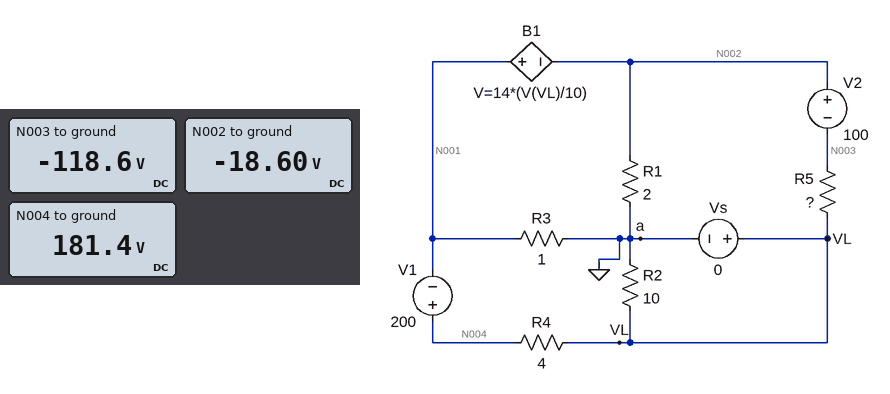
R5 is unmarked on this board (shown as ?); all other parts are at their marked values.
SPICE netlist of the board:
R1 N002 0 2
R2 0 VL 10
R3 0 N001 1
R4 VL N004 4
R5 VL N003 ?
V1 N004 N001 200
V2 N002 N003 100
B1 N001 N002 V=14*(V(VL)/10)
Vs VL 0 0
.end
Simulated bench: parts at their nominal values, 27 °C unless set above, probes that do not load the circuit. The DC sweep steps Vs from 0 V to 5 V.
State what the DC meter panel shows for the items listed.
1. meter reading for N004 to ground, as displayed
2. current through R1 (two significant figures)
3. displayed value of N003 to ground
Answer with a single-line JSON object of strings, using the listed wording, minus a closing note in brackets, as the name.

{"meter reading for N004 to ground, as displayed": "181.4 V", "current through R1": "9.3 A", "displayed value of N003 to ground": "-118.6 V"}
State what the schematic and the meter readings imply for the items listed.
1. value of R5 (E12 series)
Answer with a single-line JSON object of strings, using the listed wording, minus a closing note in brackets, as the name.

{"value of R5": "6.8 Ω"}
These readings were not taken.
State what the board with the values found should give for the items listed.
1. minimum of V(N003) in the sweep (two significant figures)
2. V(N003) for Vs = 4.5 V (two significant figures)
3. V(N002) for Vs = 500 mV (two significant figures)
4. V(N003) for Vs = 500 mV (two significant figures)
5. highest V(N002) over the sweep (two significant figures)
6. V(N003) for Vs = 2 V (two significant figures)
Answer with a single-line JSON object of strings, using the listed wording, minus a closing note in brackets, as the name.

{"minimum of V(N003) in the sweep": "-120 V", "V(N003) for Vs = 4.5 V": "-120 V", "V(N002) for Vs = 500 mV": "-19 V", "V(N003) for Vs = 500 mV": "-120 V", "highest V(N002) over the sweep": "-19 V", "V(N003) for Vs = 2 V": "-120 V"}
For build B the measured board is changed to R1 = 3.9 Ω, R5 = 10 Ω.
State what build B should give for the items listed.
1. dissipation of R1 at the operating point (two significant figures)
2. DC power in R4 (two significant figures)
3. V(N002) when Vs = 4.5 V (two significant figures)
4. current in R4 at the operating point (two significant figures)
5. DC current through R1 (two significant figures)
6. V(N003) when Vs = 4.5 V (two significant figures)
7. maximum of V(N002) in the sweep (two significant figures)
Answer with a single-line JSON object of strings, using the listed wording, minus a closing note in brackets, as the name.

{"dissipation of R1 at the operating point": "160 W", "DC power in R4": "7.7 kW", "V(N002) when Vs = 4.5 V": "-29 V", "current in R4 at the operating point": "44 A", "DC current through R1": "6.4 A", "V(N003) when Vs = 4.5 V": "-130 V", "maximum of V(N002) in the sweep": "-25 V"}
